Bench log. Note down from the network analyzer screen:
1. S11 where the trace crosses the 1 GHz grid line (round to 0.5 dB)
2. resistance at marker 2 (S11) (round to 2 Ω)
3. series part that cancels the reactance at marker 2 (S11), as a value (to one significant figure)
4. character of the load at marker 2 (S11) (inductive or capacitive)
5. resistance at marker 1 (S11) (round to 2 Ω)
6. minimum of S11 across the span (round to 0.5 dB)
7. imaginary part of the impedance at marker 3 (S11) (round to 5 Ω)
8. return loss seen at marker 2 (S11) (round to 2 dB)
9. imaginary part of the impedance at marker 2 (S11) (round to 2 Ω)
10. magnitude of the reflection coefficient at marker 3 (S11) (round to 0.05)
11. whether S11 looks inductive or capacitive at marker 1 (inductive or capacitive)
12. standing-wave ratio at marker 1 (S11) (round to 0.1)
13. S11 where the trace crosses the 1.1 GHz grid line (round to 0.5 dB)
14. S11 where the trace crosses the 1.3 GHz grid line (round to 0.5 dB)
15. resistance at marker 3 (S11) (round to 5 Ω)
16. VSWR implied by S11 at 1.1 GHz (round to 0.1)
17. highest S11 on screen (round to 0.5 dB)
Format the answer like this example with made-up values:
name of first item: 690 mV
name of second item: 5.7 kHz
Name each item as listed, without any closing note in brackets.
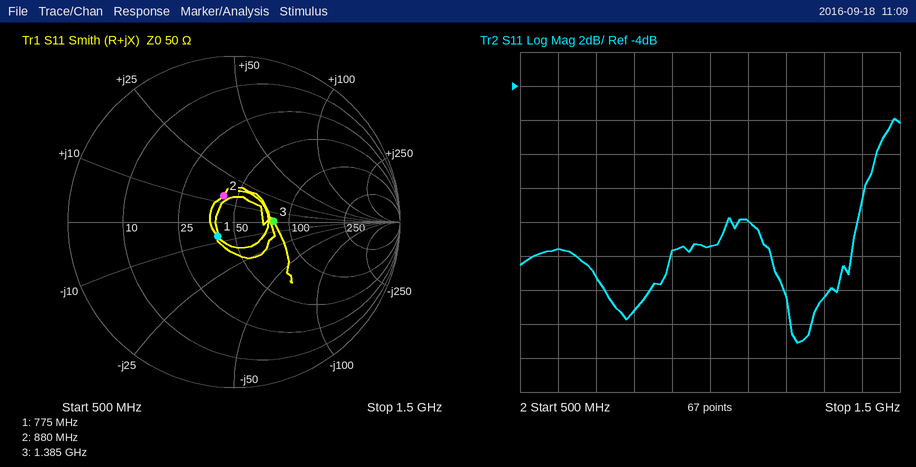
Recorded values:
S11 where the trace crosses the 1 GHz grid line: -13.5 dB
resistance at marker 2 (S11): 42 Ω
series part that cancels the reactance at marker 2 (S11), as a value: 10 pF
character of the load at marker 2 (S11): inductive
resistance at marker 1 (S11): 40 Ω
minimum of S11 across the span: -19.0 dB
imaginary part of the impedance at marker 3 (S11): 0 Ω
return loss seen at marker 2 (S11): 16 dB
imaginary part of the impedance at marker 2 (S11): +14 Ω
magnitude of the reflection coefficient at marker 3 (S11): 0.25
whether S11 looks inductive or capacitive at marker 1: capacitive
standing-wave ratio at marker 1 (S11): 1.3
S11 where the trace crosses the 1.1 GHz grid line: -12.0 dB
S11 where the trace crosses the 1.3 GHz grid line: -16.5 dB
resistance at marker 3 (S11): 80 Ω
VSWR implied by S11 at 1.1 GHz: 1.7
highest S11 on screen: -6.0 dB
